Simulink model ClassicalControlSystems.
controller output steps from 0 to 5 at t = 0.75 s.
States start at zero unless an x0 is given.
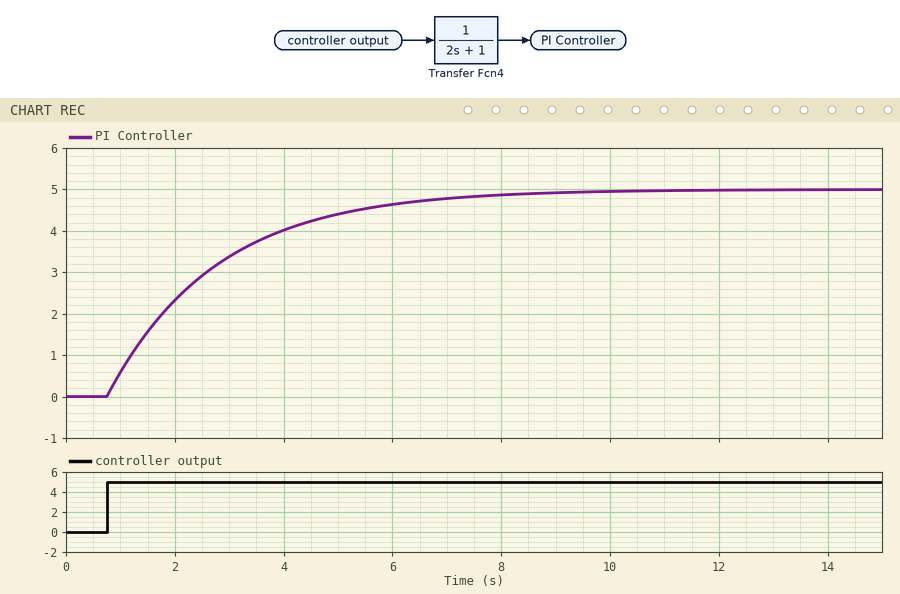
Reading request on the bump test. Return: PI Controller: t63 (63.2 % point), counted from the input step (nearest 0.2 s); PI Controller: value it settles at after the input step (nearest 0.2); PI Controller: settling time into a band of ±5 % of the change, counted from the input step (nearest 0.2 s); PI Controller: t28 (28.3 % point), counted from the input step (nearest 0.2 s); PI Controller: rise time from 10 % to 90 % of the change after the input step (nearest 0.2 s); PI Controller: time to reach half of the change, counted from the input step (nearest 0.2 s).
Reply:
2.0 s
5.0
6.0 s
0.6 s
4.4 s
1.4 s
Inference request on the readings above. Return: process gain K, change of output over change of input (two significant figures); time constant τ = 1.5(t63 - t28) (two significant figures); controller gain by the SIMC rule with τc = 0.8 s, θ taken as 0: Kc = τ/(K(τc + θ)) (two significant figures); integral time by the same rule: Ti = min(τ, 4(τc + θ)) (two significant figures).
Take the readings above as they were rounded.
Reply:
1.0
2.1 s
2.6
2.1 s
